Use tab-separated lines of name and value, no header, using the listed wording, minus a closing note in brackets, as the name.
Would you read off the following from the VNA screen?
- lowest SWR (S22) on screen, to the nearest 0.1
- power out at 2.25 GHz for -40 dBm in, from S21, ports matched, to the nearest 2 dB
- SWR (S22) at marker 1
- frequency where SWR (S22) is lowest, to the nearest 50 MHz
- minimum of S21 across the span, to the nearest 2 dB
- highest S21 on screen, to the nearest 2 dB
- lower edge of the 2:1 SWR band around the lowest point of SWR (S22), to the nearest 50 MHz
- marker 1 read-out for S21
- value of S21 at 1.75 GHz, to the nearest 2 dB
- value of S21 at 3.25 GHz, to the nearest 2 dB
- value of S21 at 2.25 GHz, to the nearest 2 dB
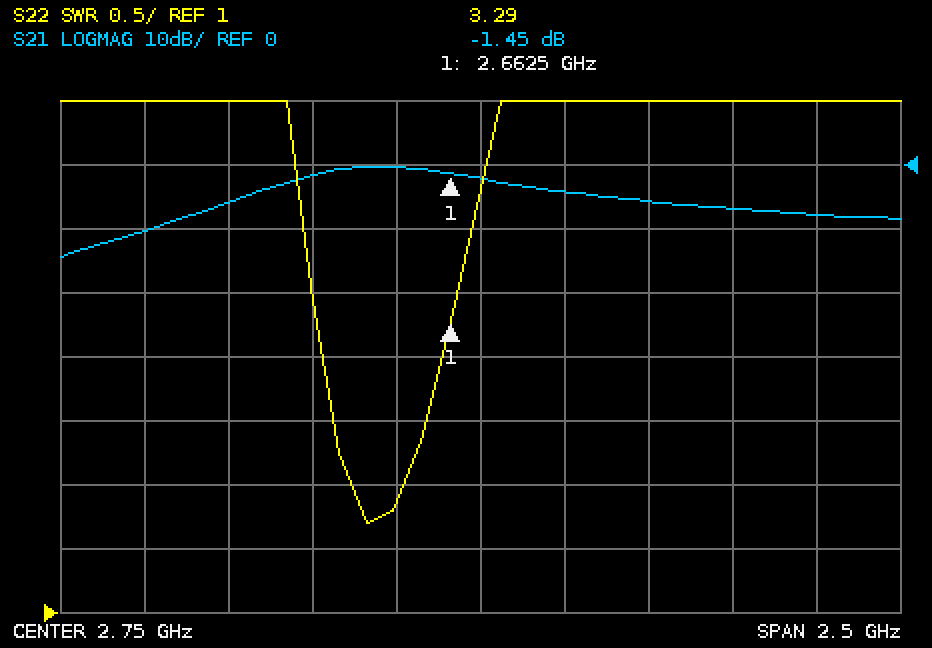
lowest SWR (S22) on screen, to the nearest 0.1	1.7
power out at 2.25 GHz for -40 dBm in, from S21, ports matched, to the nearest 2 dB	-42 dBm
SWR (S22) at marker 1	3.29
frequency where SWR (S22) is lowest, to the nearest 50 MHz	2.40 GHz
minimum of S21 across the span, to the nearest 2 dB	-14 dB
highest S21 on screen, to the nearest 2 dB	0 dB
lower edge of the 2:1 SWR band around the lowest point of SWR (S22), to the nearest 50 MHz	2.35 GHz
marker 1 read-out for S21	-1.45 dB
value of S21 at 1.75 GHz, to the nearest 2 dB	-10 dB
value of S21 at 3.25 GHz, to the nearest 2 dB	-6 dB
value of S21 at 2.25 GHz, to the nearest 2 dB	-2 dB
